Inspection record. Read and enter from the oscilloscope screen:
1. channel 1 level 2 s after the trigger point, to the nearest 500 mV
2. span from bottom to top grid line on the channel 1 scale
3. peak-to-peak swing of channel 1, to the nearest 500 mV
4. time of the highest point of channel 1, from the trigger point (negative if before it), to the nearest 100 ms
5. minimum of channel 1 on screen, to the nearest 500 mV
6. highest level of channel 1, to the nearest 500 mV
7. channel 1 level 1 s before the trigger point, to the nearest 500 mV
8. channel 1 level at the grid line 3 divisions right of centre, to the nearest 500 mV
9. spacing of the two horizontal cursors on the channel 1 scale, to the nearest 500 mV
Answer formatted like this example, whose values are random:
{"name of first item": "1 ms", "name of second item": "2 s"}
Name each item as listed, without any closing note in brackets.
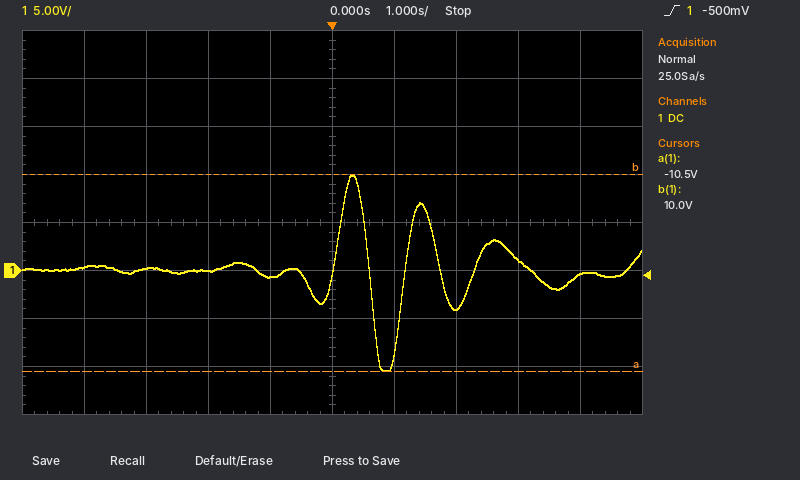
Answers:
{"channel 1 level 2 s after the trigger point, to the nearest 500 mV": "-4.0 V", "span from bottom to top grid line on the channel 1 scale": "40 V", "peak-to-peak swing of channel 1, to the nearest 500 mV": "20.5 V", "time of the highest point of channel 1, from the trigger point (negative if before it), to the nearest 100 ms": "+300 ms", "minimum of channel 1 on screen, to the nearest 500 mV": "-10.5 V", "highest level of channel 1, to the nearest 500 mV": "10.0 V", "channel 1 level 1 s before the trigger point, to the nearest 500 mV": "-500 mV", "channel 1 level at the grid line 3 divisions right of centre, to the nearest 500 mV": "1.0 V", "spacing of the two horizontal cursors on the channel 1 scale, to the nearest 500 mV": "20.5 V"}
